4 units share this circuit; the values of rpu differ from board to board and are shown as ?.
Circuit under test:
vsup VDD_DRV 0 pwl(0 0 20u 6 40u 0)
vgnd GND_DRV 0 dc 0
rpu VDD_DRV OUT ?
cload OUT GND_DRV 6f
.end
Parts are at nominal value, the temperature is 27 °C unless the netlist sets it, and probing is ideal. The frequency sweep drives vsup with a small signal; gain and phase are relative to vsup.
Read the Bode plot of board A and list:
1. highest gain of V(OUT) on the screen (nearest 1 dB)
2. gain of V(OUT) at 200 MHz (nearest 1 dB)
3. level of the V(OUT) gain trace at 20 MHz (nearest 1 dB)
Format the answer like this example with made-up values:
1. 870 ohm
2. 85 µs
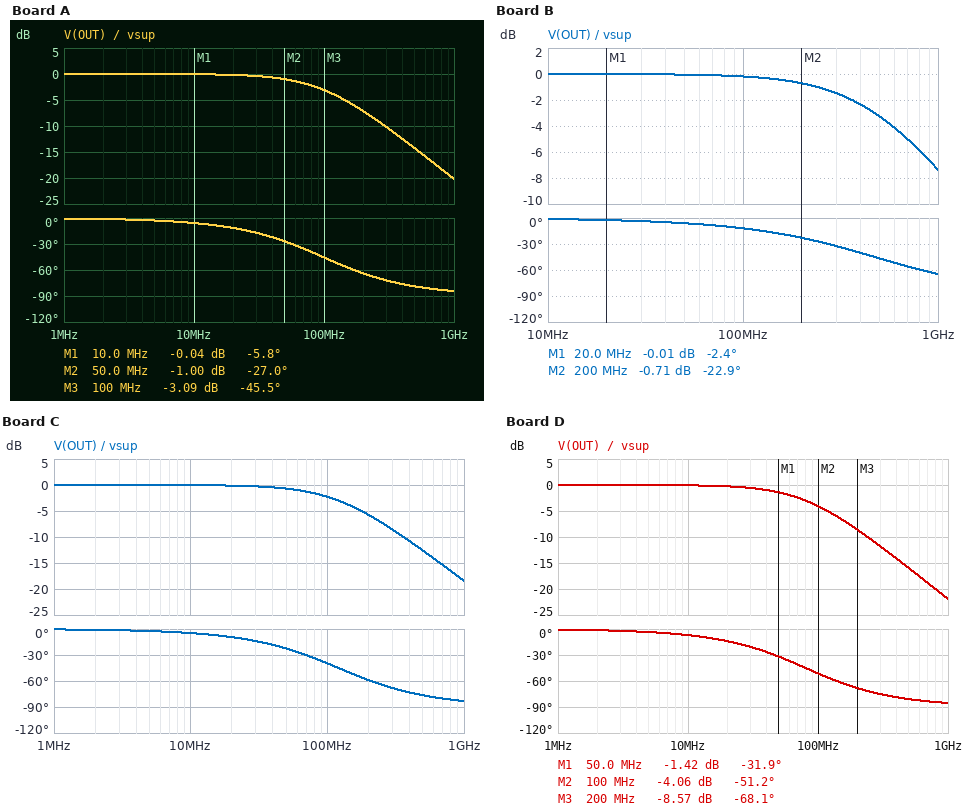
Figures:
1. 0 dB
2. -7 dB
3. 0 dB
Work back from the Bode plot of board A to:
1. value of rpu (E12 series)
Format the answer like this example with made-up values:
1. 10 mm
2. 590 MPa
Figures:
1. 270 kΩ
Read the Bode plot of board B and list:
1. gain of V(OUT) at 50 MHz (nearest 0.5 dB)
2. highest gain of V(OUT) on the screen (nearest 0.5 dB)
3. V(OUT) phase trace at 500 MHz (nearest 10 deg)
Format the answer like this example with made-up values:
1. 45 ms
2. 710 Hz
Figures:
1. 0 dB
2. 0 dB
3. -50 deg
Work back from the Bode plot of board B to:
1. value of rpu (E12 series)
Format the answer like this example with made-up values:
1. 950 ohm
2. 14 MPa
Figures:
1. 56 kΩ
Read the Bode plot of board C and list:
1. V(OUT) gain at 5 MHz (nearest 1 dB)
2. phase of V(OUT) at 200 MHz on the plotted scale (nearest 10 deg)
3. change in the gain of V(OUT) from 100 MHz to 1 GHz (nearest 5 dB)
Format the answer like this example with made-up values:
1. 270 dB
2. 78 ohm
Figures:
1. 0 dB
2. -60 deg
3. -15 dB
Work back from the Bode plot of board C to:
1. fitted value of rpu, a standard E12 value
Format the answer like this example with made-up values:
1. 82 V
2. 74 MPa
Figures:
1. 220 kΩ
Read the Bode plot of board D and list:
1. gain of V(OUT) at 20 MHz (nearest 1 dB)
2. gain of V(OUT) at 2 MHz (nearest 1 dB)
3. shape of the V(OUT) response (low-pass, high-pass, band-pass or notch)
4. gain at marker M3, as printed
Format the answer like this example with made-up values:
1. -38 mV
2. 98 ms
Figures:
1. 0 dB
2. 0 dB
3. low-pass
4. -8.57 dB
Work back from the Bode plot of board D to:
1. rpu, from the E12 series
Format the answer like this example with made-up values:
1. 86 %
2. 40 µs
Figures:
1. 330 kΩ
